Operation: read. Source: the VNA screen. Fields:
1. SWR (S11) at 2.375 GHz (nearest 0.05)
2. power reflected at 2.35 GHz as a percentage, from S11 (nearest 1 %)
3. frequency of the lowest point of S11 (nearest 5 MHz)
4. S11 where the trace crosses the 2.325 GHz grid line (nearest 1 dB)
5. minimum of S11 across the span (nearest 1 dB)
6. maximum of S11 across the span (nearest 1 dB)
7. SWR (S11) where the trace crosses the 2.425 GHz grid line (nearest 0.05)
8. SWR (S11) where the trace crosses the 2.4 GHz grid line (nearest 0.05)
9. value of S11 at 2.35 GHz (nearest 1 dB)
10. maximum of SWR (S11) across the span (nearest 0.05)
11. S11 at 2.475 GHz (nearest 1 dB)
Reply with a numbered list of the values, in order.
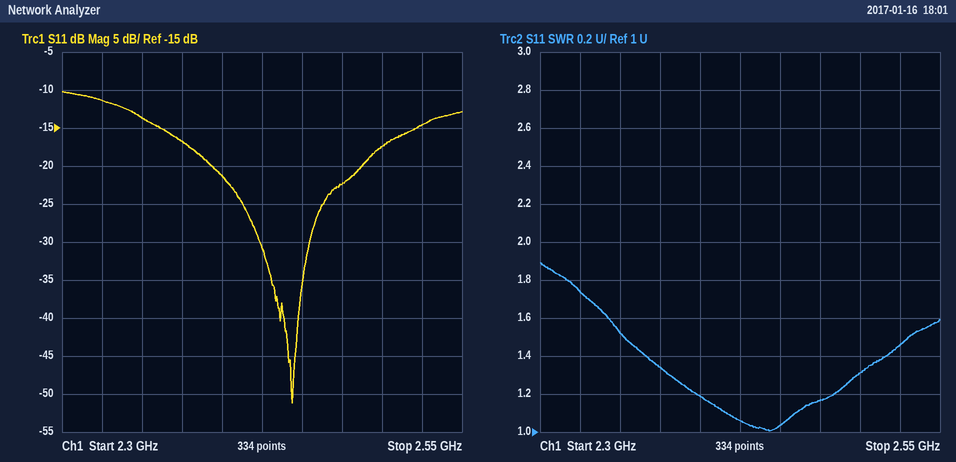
1. 1.35
2. 4 %
3. 2.445 GHz
4. -11 dB
5. -51 dB
6. -10 dB
7. 1.05
8. 1.20
9. -14 dB
10. 1.90
11. -22 dB
